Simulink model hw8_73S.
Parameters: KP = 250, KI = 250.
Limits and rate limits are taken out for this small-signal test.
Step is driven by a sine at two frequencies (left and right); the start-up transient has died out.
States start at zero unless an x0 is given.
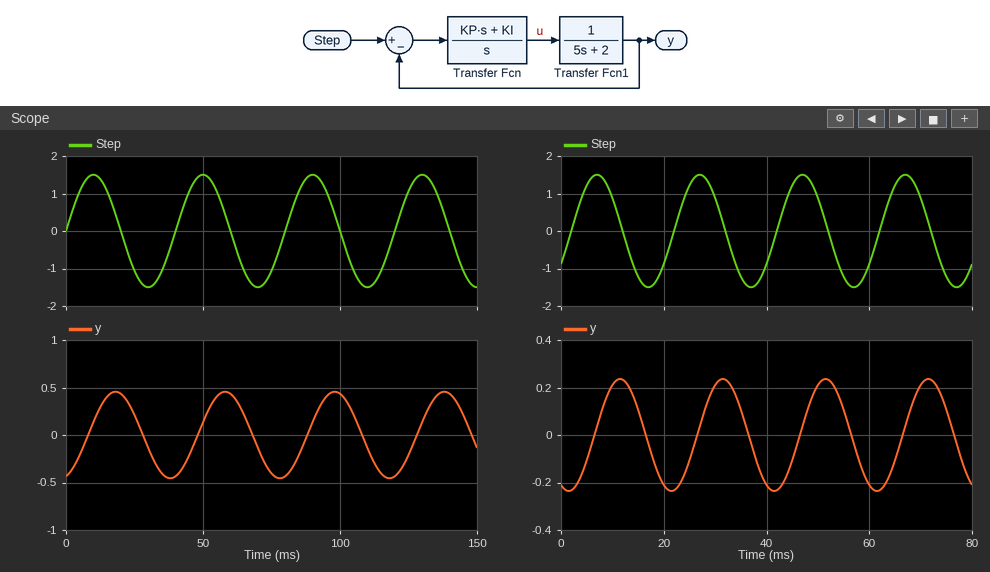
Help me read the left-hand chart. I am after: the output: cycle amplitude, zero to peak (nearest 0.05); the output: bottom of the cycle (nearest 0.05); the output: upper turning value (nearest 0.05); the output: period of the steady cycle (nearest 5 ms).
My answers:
0.45
-0.45
0.45
40 ms
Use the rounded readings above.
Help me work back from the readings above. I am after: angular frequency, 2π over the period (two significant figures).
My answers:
0.16 rad/ms
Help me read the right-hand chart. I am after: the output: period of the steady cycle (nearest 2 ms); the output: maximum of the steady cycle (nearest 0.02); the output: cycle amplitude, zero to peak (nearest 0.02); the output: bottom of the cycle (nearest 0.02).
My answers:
20 ms
0.24
0.24
-0.24
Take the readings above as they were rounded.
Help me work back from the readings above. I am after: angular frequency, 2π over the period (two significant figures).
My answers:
0.31 rad/ms
